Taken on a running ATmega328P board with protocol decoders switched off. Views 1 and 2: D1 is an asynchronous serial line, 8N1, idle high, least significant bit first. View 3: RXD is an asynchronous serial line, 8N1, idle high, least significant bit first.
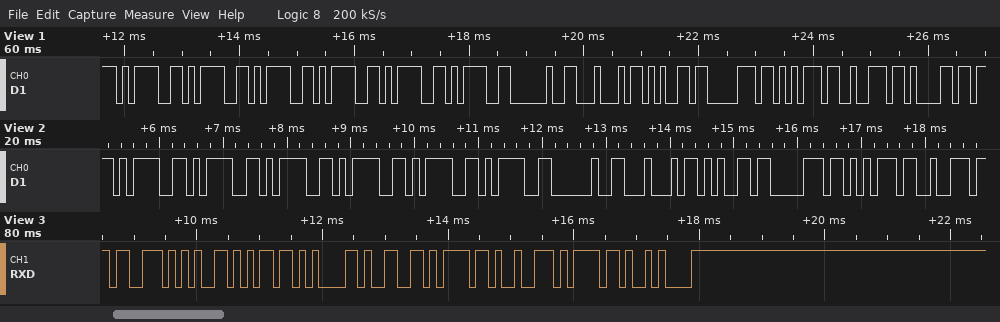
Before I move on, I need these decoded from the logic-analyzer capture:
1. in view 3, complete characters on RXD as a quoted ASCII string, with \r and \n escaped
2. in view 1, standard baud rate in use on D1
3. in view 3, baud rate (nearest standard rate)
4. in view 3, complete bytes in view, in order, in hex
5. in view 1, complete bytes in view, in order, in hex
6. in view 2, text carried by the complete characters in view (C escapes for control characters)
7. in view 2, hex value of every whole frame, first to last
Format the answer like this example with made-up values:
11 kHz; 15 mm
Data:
"semaforo\n"; 9600 baud; 9600 baud; 0x73 0x65 0x6D 0x61 0x66 0x6F 0x72 0x6F 0x0A; 3D 3D 3D 3D 3D 3D 20 44 65 70 75 72 61; "====== Depur"; 0x3D 0x3D 0x3D 0x3D 0x3D 0x3D 0x20 0x44 0x65 0x70 0x75 0x72
